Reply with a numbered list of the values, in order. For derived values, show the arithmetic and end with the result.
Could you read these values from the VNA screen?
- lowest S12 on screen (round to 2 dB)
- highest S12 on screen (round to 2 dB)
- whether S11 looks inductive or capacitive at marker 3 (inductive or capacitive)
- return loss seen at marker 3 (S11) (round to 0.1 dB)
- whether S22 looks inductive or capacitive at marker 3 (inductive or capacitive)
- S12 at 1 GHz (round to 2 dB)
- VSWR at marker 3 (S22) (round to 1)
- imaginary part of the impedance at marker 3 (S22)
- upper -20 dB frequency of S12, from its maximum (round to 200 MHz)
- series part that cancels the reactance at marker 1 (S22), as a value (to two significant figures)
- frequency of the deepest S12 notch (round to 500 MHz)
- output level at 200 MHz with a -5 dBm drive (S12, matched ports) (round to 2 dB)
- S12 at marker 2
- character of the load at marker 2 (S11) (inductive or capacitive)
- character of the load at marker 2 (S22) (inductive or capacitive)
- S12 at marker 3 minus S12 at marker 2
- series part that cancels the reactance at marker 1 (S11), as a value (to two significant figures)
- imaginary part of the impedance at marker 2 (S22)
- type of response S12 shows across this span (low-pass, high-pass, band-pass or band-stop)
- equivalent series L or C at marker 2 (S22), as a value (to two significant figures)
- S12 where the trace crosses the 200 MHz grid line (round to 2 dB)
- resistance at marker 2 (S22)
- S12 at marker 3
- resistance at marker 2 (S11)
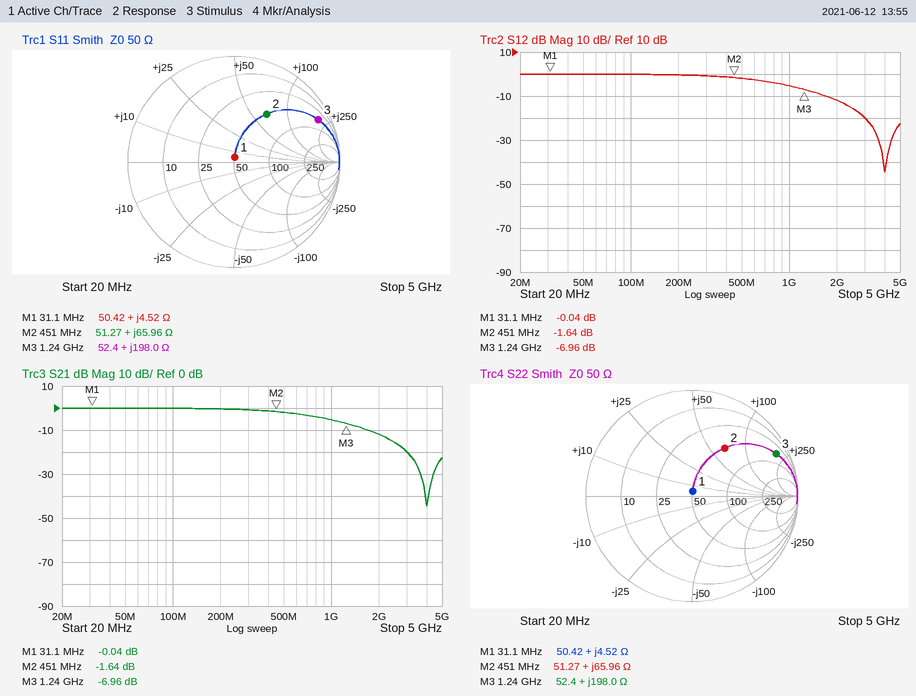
1. -44 dB
2. 0 dB
3. inductive
4. 1.0 dB
5. inductive
6. -6 dB
7. 17
8. +198.0 Ω
9. 3.0 GHz
10. C = 1/(2π × 31.1 MHz × 4.52 Ω) ≈ 1.1 nF
11. 4.0 GHz
12. -5 dBm + (0 dB) = -6 dBm
13. -1.64 dB
14. inductive
15. inductive
16. -6.96 − (-1.64) = -5.32 dB
17. C = 1/(2π × 31.1 MHz × 4.52 Ω) ≈ 1.1 nF
18. +65.96 Ω
19. low-pass
20. L = 65.96 Ω/(2π × 451 MHz) ≈ 23 nH
21. 0 dB
22. 51.27 Ω
23. -6.96 dB
24. 51.27 Ω
